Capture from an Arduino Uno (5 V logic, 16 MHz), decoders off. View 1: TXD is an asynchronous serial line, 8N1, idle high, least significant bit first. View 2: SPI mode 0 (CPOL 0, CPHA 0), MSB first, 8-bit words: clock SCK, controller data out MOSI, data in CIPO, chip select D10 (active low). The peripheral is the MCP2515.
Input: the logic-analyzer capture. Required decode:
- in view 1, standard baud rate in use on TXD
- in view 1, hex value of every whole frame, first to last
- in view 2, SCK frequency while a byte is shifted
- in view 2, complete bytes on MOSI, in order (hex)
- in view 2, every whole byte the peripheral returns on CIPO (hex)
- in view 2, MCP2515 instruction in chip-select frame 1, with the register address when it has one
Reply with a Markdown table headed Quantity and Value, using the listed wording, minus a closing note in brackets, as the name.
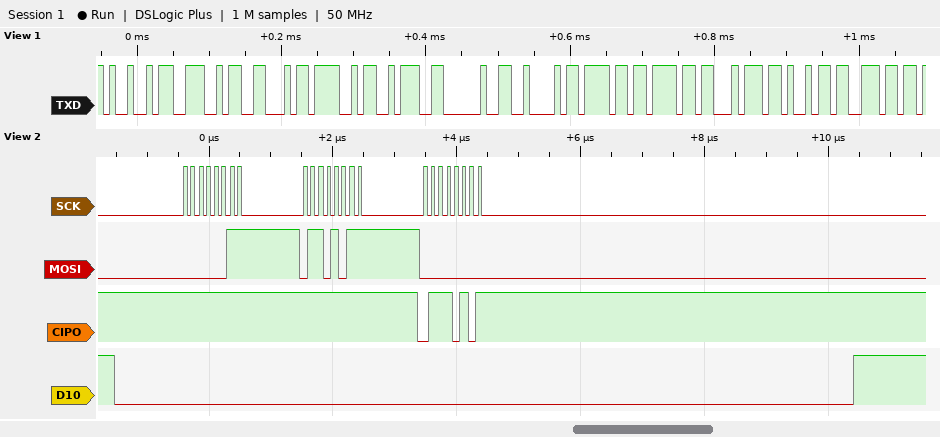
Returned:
| Quantity | Value |
|---|---|
| in view 1, standard baud rate in use on TXD | 115200 baud |
| in view 1, hex value of every whole frame, first to last | 49 4E 46 4F 3A 20 42 6F 6F 74 69 6E |
| in view 2, SCK frequency while a byte is shifted | 8 MHz |
| in view 2, complete bytes on MOSI, in order | 03 6B 00 |
| in view 2, every whole byte the peripheral returns on CIPO | FF FF 75 |
| in view 2, MCP2515 instruction in chip-select frame 1, with the register address when it has one | READ 0x6B |
